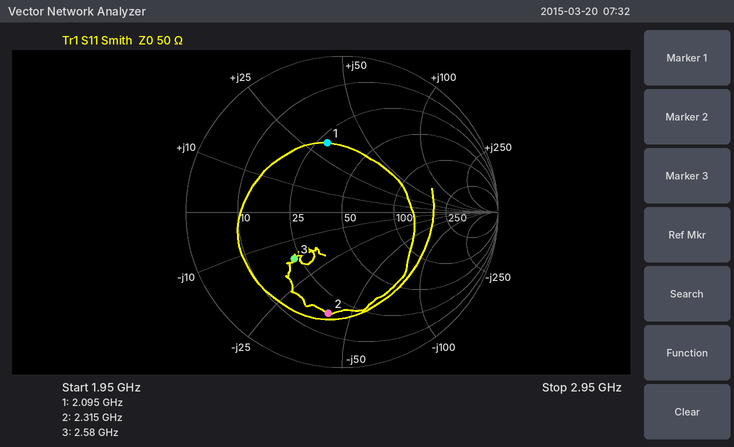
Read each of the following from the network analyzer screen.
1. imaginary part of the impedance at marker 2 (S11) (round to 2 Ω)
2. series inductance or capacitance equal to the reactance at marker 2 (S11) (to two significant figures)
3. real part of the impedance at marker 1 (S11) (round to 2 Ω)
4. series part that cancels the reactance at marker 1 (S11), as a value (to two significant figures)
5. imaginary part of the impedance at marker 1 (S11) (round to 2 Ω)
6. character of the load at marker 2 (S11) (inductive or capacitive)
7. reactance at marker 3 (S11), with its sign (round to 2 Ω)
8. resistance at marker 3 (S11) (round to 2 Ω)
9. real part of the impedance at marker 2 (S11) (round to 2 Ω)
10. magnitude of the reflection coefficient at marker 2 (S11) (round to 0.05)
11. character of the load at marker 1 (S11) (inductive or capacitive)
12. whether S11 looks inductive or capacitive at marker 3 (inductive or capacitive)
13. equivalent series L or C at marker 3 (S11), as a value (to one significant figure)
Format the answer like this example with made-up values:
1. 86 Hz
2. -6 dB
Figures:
1. -40 Ω
2. 1.7 pF
3. 28 Ω
4. 2.4 pF
5. +32 Ω
6. capacitive
7. -16 Ω
8. 22 Ω
9. 18 Ω
10. 0.65
11. inductive
12. capacitive
13. 4 pF
